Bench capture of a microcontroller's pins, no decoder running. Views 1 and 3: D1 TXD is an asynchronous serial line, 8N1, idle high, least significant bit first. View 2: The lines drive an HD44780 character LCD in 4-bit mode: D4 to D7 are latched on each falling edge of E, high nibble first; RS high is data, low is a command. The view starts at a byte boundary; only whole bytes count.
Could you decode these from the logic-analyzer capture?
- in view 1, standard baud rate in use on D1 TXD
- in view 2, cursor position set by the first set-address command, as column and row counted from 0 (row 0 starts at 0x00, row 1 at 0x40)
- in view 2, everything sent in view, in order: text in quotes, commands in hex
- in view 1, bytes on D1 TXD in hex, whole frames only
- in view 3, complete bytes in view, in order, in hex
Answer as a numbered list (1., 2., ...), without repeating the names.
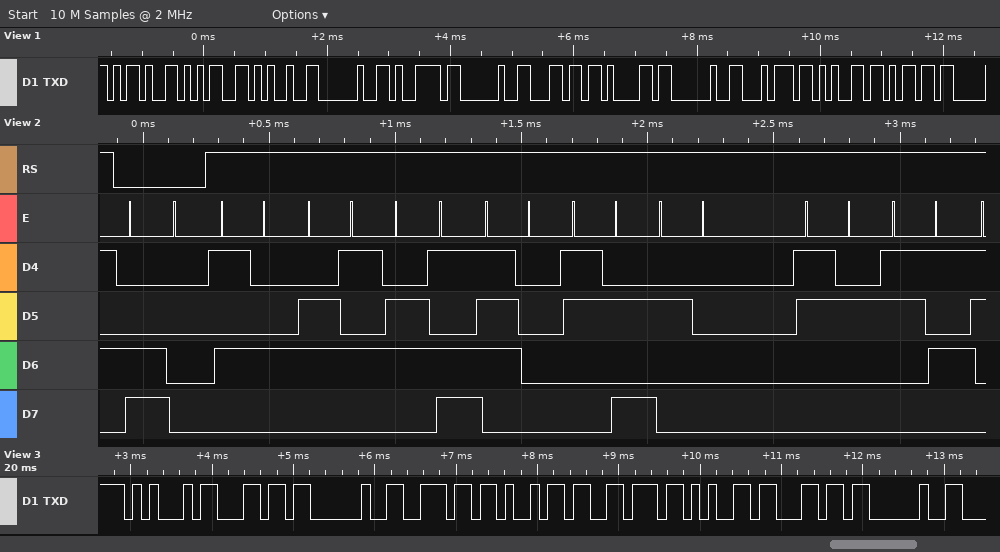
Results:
1. 9600 baud
2. column 0, row 1
3. 0xC0 "Temp: 25"
4. 2D 35 25 20 79 20 6C 61 20 74 65 6D
5. 45 6C 20 6E 69 76 65 6C 20
